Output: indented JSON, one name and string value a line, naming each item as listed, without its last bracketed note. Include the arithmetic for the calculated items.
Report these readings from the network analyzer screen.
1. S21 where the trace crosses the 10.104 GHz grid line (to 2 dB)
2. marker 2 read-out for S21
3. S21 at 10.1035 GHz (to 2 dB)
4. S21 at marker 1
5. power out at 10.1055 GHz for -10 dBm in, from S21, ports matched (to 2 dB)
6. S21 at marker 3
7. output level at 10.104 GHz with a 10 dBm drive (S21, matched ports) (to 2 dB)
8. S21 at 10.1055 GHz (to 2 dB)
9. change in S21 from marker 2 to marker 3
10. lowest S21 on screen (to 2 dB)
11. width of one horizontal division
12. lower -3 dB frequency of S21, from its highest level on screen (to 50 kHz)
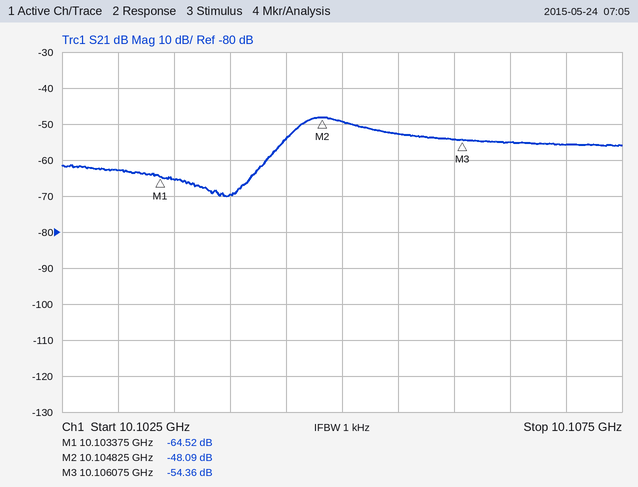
{
  "S21 where the trace crosses the 10.104 GHz grid line": "-70 dB",
  "marker 2 read-out for S21": "-48.09 dB",
  "S21 at 10.1035 GHz": "-66 dB",
  "S21 at marker 1": "-64.52 dB",
  "power out at 10.1055 GHz for -10 dBm in, from S21, ports matched": "-10 dBm + (-52 dB) = -62 dBm",
  "S21 at marker 3": "-54.36 dB",
  "output level at 10.104 GHz with a 10 dBm drive (S21, matched ports)": "10 dBm + (-70 dB) = -60 dBm",
  "S21 at 10.1055 GHz": "-52 dB",
  "change in S21 from marker 2 to marker 3": "-54.36 − (-48.09) = -6.27 dB",
  "lowest S21 on screen": "-70 dB",
  "width of one horizontal division": "500 kHz",
  "lower -3 dB frequency of S21, from its highest level on screen": "10.10460 GHz"
}
